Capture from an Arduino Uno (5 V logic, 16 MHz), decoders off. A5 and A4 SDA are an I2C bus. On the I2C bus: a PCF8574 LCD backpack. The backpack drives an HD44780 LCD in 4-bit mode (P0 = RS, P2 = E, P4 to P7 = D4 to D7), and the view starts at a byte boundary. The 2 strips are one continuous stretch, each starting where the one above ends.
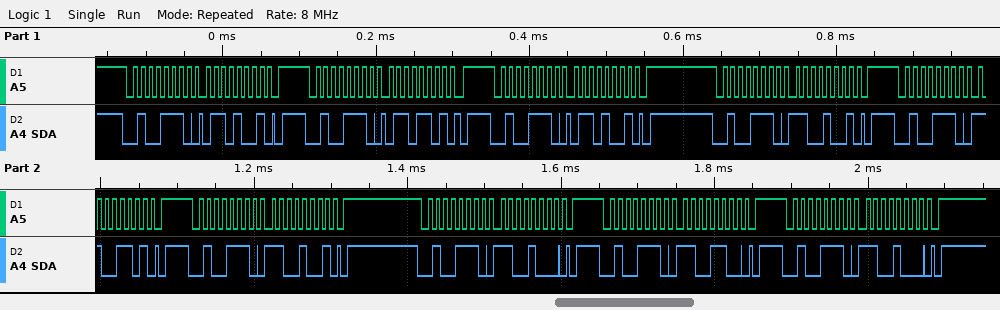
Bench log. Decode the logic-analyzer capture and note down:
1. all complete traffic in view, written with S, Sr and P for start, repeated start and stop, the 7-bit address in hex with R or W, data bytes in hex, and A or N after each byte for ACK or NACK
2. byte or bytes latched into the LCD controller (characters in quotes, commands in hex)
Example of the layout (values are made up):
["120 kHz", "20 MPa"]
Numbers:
["S 27W A 69 A P S 27W A 6D A P S 27W A 69 A P S 27W A C9 A P S 27W A CD A P S 27W A C9 A P S 27W A C8 A P S 27W A CC A P S 27W A C8 A P", "'l'"]
